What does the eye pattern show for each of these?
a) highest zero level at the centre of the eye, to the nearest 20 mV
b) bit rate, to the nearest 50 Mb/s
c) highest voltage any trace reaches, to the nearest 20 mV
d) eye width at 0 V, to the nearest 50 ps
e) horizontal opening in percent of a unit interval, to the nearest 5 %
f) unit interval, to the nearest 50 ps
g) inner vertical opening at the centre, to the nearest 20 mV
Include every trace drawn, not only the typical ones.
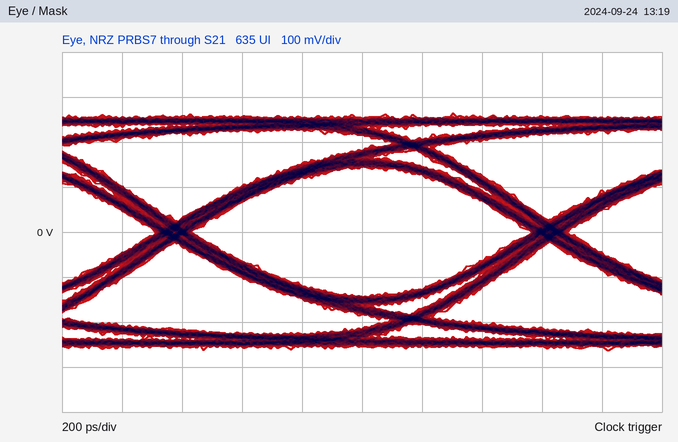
-140 mV
800 Mb/s
260 mV
1.15 ns
90 %
1.25 ns
280 mV
